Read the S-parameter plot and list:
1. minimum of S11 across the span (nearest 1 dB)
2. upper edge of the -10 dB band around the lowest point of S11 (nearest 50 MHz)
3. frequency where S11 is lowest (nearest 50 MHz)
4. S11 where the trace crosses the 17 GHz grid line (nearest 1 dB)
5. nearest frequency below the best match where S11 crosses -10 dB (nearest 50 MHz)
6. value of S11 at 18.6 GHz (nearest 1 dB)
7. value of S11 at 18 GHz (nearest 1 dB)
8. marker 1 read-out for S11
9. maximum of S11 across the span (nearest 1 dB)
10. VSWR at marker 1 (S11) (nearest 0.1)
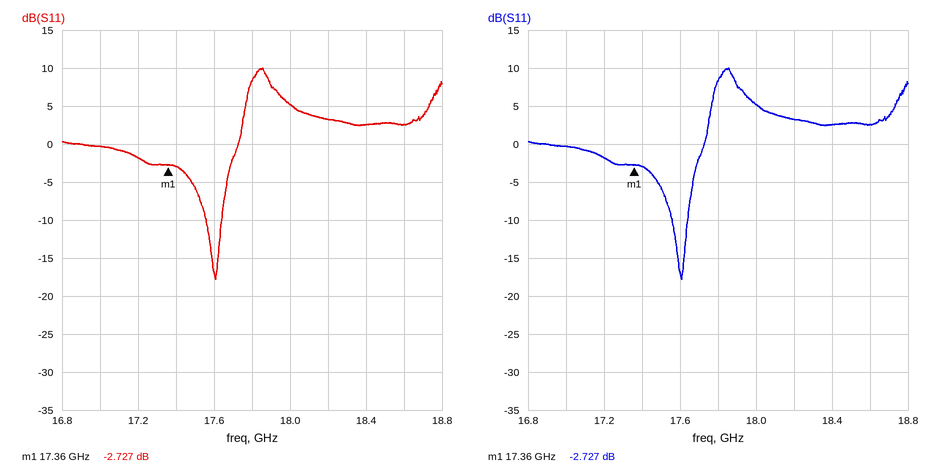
-18 dB
17.65 GHz
17.60 GHz
0 dB
17.55 GHz
3 dB
5 dB
-2.727 dB
10 dB
6.4
